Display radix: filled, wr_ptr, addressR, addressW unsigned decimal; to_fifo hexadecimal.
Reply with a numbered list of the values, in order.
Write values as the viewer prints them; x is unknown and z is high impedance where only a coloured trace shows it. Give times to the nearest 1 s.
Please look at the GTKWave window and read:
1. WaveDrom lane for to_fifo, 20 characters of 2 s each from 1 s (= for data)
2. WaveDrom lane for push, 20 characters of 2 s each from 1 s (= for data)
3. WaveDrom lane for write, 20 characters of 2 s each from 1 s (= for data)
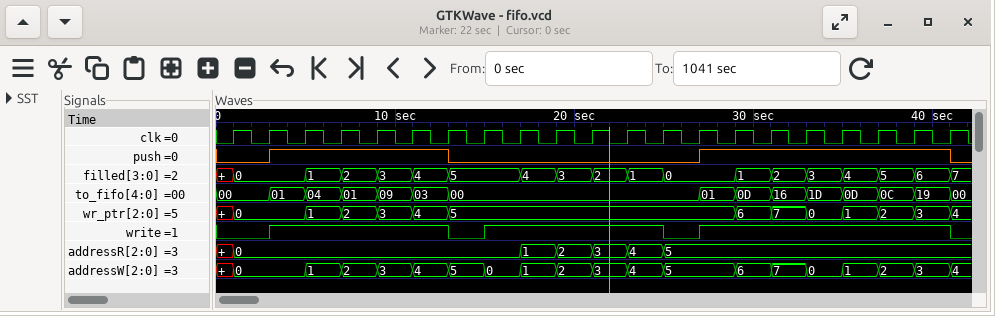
1. {name: 'to_fifo', wave: '=======......=======', data: '00 01 04 01 09 03 00 01 0D 16 1D 0D 0C 19'}
2. {name: 'push', wave: '01....0......1......'}
3. {name: 'write', wave: '01....01....01......'}
